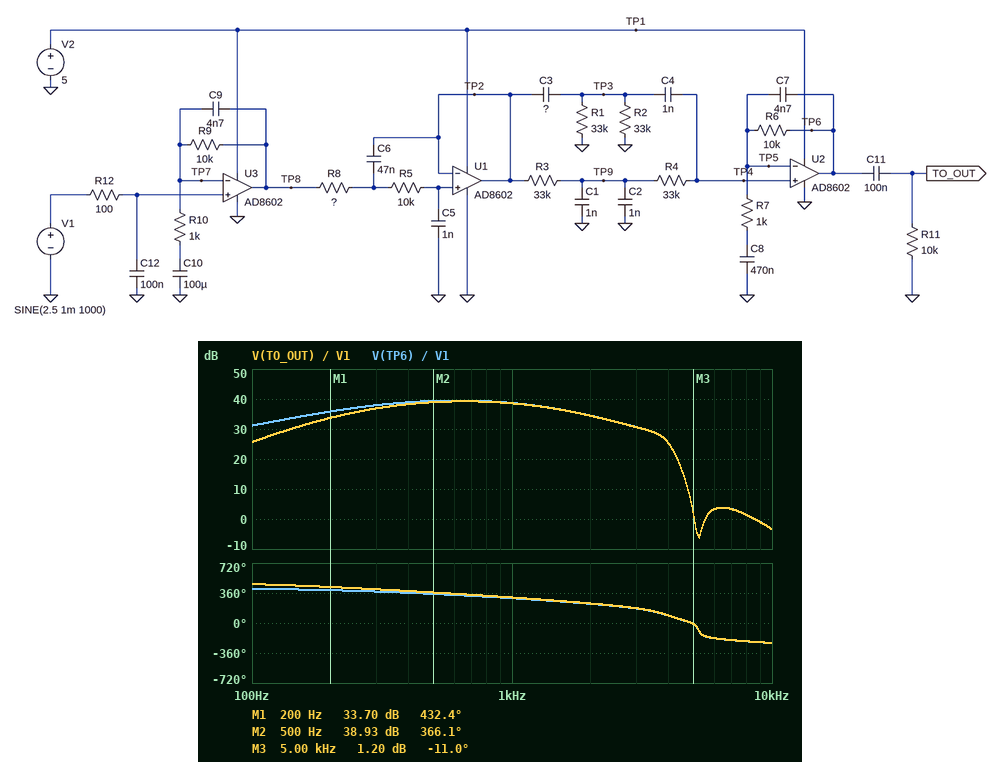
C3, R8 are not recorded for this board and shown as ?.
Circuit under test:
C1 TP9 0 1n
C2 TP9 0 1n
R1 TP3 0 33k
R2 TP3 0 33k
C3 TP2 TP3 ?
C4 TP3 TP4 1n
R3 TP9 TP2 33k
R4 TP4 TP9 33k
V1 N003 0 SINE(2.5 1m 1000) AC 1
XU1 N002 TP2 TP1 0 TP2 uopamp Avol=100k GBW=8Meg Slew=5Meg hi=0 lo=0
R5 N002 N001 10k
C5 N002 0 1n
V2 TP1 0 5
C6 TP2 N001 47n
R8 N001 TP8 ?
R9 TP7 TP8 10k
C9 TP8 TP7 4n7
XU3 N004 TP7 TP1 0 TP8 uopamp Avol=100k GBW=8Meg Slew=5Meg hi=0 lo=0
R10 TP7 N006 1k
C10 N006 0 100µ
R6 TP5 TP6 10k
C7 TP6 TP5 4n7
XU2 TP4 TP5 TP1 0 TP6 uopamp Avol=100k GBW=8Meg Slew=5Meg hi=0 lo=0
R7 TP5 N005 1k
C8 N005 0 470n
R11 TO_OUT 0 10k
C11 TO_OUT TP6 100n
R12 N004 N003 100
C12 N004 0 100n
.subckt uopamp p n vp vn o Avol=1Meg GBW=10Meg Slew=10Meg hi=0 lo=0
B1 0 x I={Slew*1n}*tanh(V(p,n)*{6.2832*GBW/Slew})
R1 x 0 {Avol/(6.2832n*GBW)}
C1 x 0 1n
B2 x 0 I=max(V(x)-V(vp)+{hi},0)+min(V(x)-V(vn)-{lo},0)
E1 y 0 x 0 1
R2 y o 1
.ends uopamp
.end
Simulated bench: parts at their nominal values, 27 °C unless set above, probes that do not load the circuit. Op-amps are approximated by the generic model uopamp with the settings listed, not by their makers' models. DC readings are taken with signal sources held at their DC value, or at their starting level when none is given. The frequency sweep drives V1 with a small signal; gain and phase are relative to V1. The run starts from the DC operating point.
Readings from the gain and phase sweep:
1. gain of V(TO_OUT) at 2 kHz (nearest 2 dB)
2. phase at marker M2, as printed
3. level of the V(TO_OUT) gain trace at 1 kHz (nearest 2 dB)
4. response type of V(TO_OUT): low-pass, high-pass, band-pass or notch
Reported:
34 dB
366.1 deg
38 dB
band-pass
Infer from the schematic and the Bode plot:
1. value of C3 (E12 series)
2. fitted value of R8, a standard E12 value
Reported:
820 pF
3.3 kΩ
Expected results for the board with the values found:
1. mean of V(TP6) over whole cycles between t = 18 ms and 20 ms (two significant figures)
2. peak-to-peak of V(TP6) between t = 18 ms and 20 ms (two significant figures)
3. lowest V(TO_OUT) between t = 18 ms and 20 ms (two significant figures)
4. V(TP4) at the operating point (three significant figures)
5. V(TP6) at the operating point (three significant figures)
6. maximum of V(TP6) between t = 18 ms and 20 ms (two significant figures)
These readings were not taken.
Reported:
2.5 V
170 mV
-85 mV
2.50 V
2.50 V
2.6 V
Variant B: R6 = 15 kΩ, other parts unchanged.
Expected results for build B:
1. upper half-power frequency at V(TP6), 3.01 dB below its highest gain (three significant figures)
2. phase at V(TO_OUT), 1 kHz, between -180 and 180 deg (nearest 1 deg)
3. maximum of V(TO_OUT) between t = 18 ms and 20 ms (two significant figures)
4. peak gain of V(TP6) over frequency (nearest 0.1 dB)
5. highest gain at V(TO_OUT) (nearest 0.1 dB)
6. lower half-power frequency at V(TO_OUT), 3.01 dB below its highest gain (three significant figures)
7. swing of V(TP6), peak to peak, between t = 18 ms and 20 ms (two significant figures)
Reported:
1.41 kHz
-60 deg
120 mV
42.6 dB
42.3 dB
267 Hz
240 mV
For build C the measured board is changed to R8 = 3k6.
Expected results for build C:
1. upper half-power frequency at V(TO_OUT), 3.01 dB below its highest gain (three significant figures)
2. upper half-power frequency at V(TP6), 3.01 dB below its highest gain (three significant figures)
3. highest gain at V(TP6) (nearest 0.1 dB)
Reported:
1.62 kHz
1.57 kHz
39.5 dB
